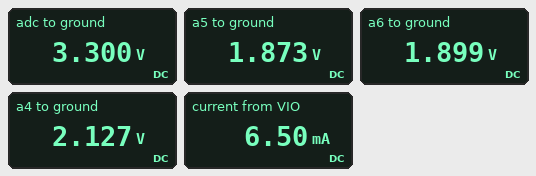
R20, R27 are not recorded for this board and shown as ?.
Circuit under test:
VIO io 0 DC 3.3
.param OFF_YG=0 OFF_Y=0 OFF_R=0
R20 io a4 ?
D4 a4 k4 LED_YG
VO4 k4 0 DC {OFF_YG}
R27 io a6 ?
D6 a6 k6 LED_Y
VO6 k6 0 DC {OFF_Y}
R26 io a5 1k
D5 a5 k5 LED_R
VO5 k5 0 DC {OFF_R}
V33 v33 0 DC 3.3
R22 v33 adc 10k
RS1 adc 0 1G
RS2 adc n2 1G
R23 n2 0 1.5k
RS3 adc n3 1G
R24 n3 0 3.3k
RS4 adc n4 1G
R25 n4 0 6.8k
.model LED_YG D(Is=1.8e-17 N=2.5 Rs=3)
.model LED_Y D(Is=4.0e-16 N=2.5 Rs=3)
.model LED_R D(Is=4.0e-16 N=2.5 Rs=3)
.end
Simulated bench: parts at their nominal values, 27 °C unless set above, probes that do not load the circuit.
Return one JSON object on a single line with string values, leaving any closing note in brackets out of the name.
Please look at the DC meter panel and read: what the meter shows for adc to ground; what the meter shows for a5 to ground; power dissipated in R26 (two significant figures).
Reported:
{"what the meter shows for adc to ground": "3.300 V", "what the meter shows for a5 to ground": "1.873 V", "power dissipated in R26": "2.0 mW"}
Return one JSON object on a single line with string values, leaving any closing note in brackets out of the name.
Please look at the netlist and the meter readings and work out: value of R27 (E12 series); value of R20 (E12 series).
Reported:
{"value of R27": "680 Ω", "value of R20": "390 Ω"}
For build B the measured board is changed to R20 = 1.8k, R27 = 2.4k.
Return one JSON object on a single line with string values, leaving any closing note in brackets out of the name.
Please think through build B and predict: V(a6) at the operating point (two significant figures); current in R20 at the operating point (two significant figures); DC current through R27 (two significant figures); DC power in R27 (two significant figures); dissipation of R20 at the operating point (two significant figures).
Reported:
{"V(a6) at the operating point": "1.8 V", "current in R20 at the operating point": "710 µA", "DC current through R27": "620 µA", "DC power in R27": "920 µW", "dissipation of R20 at the operating point": "900 µW"}
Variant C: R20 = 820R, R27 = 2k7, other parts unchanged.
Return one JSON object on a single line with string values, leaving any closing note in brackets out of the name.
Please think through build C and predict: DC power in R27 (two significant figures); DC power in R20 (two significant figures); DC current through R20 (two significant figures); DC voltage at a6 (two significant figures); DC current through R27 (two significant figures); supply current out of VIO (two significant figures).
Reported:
{"DC power in R27": "820 µW", "DC power in R20": "1.8 mW", "DC current through R20": "1.5 mA", "DC voltage at a6": "1.8 V", "DC current through R27": "550 µA", "supply current out of VIO": "3.5 mA"}
